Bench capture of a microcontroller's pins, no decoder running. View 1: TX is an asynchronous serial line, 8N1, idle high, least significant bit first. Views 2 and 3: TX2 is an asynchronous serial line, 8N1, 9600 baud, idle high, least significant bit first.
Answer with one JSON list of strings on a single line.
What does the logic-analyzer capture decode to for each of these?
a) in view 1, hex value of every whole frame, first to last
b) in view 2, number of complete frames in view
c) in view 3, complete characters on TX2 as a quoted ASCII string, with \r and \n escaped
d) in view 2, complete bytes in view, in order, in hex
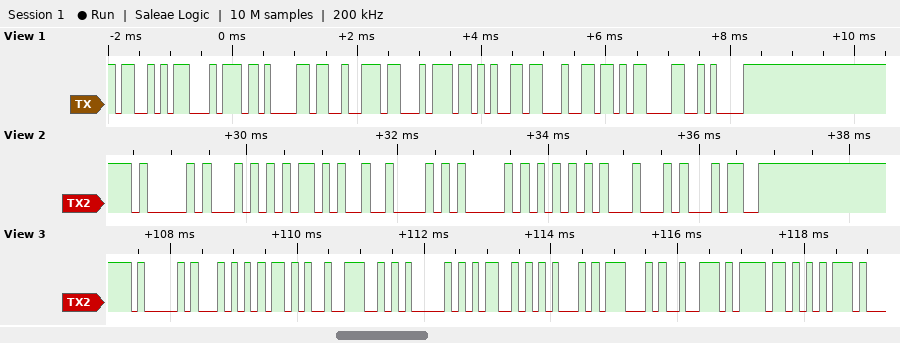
["53 74 61 72 74 65 64 0D 0A", "8", "\"AT+NAMEGrou\"", "0x41 0x54 0x2B 0x42 0x41 0x55 0x44 0x34"]
